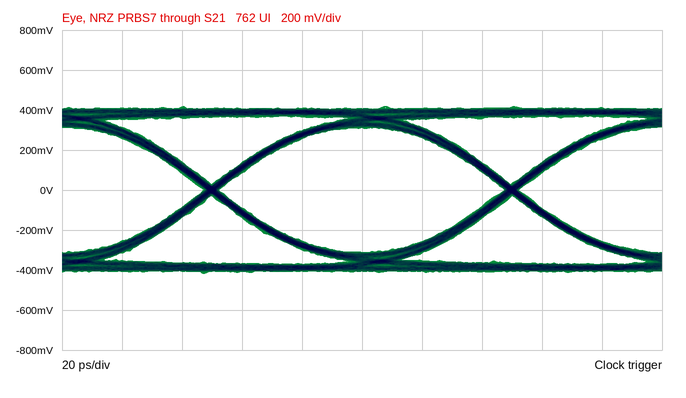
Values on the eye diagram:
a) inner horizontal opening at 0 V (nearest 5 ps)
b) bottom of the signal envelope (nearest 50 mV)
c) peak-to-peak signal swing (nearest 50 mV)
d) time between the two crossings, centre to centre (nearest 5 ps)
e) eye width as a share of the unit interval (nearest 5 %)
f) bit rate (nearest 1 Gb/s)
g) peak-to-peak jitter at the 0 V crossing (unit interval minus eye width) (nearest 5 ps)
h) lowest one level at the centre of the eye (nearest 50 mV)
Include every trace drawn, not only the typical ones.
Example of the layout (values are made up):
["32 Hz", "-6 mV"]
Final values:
["95 ps", "-400 mV", "850 mV", "100 ps", "95 %", "10 Gb/s", "5 ps", "300 mV"]
